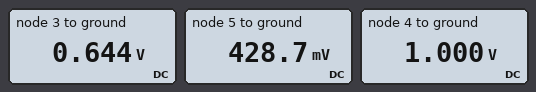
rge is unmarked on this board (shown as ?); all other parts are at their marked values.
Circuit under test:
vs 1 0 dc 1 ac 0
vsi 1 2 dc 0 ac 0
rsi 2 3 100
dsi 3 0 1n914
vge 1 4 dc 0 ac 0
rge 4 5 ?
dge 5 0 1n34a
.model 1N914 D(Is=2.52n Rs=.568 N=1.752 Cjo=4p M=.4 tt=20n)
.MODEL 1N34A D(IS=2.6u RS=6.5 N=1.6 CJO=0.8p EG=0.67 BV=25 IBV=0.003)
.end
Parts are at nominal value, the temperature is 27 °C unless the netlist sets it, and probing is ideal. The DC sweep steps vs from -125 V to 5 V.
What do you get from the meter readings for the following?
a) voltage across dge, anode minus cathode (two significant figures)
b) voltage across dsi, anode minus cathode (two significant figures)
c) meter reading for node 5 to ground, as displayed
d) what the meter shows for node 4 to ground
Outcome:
430 mV
640 mV
428.7 mV
1.000 V
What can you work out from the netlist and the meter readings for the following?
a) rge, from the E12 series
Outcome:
47 Ω
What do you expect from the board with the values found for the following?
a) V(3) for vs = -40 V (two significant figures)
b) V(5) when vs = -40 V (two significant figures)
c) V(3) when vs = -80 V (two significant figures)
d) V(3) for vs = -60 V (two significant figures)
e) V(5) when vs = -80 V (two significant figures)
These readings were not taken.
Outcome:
-40 V
-27 V
-80 V
-60 V
-32 V
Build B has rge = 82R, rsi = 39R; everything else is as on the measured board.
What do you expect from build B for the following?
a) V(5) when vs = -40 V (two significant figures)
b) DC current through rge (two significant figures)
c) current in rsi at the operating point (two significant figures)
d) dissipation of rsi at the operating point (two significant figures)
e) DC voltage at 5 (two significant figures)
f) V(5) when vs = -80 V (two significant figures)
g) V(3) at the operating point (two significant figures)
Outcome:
-26 V
7.6 mA
8.1 mA
2.6 mW
380 mV
-29 V
680 mV
